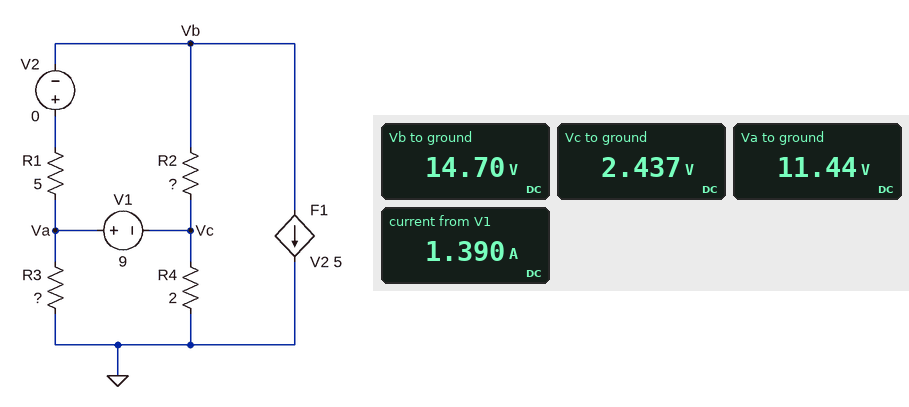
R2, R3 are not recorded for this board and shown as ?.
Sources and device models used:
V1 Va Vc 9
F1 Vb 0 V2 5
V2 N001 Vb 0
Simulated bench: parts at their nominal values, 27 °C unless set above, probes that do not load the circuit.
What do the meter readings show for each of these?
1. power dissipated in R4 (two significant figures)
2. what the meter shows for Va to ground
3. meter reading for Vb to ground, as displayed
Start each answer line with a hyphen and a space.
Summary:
- 3.0 W
- 11.44 V
- 14.70 V
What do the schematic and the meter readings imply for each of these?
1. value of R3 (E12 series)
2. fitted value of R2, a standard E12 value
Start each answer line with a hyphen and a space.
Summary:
- 5.6 Ω
- 4.7 Ω
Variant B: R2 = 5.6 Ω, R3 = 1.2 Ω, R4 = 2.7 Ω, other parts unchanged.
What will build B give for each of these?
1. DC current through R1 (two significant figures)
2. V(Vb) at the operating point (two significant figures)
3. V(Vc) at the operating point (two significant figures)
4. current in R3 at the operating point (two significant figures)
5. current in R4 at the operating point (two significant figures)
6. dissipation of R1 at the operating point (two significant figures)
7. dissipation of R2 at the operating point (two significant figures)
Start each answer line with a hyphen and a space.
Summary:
- 520 mA
- 7.5 V
- -4.1 V
- 4.1 A
- 1.5 A
- 1.3 W
- 24 W
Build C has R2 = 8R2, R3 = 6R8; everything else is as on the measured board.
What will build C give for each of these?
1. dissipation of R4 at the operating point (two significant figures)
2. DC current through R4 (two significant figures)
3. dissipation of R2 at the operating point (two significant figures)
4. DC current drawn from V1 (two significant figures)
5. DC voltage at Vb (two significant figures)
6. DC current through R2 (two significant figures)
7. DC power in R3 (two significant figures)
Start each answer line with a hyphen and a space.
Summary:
- 100 mW
- 230 mA
- 14 W
- 1.1 A
- 11 V
- 1.3 A
- 13 W
